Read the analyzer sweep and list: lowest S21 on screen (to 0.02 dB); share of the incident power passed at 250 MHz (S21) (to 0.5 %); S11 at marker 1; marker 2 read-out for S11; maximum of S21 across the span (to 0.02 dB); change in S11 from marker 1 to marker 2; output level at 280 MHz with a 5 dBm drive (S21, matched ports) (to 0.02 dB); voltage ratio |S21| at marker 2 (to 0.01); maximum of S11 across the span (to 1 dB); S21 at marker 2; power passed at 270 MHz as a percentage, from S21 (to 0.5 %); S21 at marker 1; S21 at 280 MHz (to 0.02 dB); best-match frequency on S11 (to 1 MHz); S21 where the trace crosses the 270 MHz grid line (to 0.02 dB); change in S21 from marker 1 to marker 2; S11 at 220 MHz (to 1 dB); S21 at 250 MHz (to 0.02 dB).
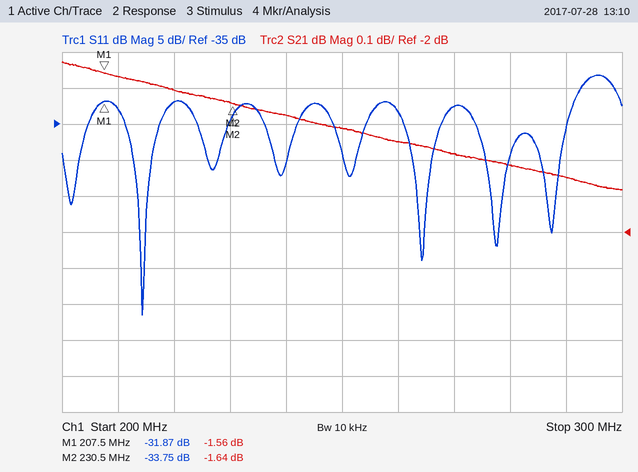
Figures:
-1.88 dB
67.5 %
-31.87 dB
-33.75 dB
-1.52 dB
-1.88 dB
3.18 dBm
0.83
-28 dB
-1.64 dB
66.5 %
-1.56 dB
-1.82 dB
214 MHz
-1.78 dB
-0.08 dB
-32 dB
-1.72 dB
